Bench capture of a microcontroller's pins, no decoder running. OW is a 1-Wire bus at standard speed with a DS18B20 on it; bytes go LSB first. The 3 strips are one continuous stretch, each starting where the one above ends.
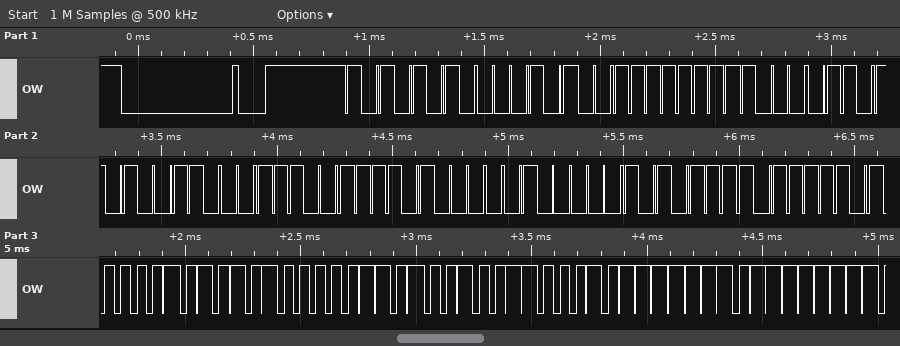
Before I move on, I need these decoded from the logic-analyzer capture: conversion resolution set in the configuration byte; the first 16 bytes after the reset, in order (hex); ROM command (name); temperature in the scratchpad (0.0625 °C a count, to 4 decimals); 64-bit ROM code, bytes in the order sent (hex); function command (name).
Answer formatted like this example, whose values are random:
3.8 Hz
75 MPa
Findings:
12 bits
55 28 FF 61 65 9C 17 04 F5 BE 50 05 4B 46 7F FF
Match ROM
85.0000 °C
28 FF 61 65 9C 17 04 F5
Read Scratchpad
